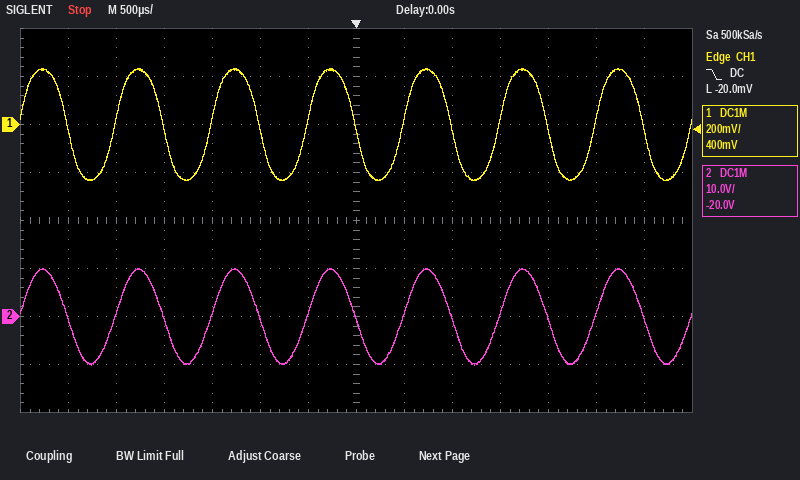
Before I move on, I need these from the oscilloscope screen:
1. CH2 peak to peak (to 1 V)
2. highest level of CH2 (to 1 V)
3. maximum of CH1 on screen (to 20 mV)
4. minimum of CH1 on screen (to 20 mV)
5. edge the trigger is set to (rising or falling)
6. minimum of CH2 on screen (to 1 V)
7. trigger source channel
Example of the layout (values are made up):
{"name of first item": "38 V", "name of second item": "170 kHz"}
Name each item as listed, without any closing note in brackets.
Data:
{"CH2 peak to peak": "20 V", "highest level of CH2": "10 V", "maximum of CH1 on screen": "240 mV", "minimum of CH1 on screen": "-240 mV", "edge the trigger is set to": "falling", "minimum of CH2 on screen": "-10 V", "trigger source channel": "CH1"}
